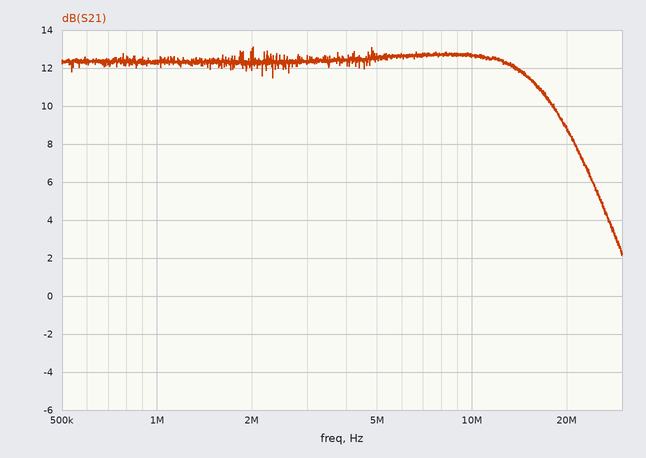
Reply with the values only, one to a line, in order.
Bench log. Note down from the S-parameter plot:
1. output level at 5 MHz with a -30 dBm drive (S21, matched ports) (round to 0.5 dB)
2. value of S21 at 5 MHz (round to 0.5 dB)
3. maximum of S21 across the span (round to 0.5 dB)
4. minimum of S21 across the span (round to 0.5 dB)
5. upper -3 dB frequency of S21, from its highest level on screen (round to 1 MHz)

-17.5 dBm
12.5 dB
13.0 dB
2.0 dB
18 MHz
